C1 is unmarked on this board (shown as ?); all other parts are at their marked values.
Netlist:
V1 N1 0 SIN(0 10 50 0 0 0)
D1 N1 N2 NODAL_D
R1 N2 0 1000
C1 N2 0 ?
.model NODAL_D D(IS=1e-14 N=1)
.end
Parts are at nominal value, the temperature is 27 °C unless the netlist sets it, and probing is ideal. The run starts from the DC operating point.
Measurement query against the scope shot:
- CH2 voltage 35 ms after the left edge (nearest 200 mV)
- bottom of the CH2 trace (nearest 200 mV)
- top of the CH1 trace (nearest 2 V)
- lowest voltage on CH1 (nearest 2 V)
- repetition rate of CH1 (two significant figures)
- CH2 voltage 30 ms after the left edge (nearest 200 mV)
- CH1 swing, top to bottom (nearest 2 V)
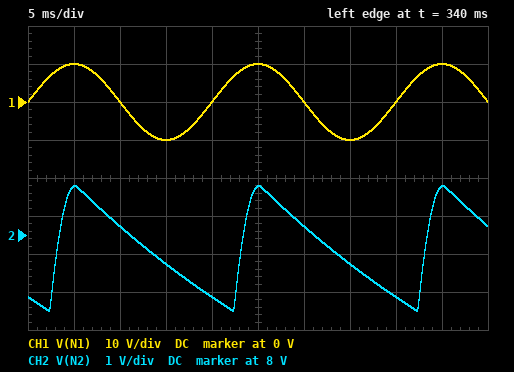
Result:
7.2 V
6.0 V
10 V
-10 V
50 Hz
8.2 V
20 V
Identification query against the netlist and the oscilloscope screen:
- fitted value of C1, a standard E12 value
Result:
39 µF
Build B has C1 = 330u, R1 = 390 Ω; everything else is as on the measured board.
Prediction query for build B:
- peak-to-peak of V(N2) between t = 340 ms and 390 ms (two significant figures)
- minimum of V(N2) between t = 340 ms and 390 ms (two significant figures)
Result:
1.2 V
8.0 V
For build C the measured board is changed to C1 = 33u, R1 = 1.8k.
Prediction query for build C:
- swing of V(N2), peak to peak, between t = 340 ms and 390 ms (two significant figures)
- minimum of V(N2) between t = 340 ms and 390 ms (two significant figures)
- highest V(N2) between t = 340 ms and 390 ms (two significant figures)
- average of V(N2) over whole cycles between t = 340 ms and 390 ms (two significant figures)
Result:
2.4 V
6.9 V
9.3 V
8.1 V
